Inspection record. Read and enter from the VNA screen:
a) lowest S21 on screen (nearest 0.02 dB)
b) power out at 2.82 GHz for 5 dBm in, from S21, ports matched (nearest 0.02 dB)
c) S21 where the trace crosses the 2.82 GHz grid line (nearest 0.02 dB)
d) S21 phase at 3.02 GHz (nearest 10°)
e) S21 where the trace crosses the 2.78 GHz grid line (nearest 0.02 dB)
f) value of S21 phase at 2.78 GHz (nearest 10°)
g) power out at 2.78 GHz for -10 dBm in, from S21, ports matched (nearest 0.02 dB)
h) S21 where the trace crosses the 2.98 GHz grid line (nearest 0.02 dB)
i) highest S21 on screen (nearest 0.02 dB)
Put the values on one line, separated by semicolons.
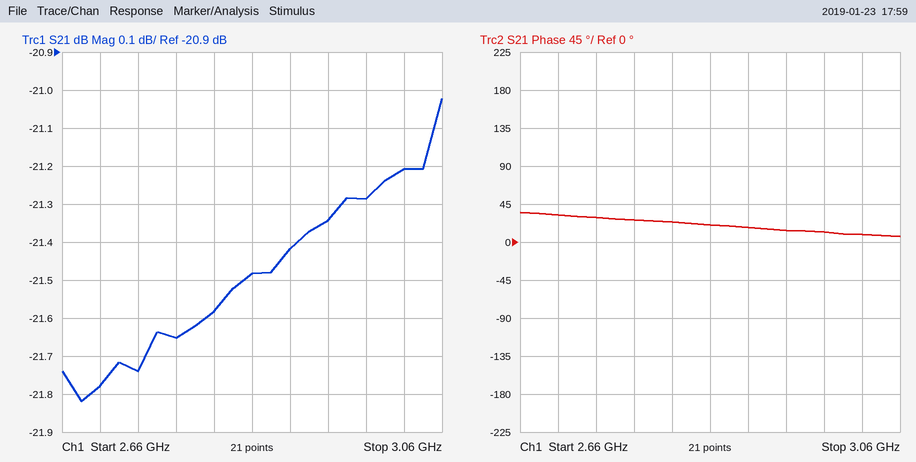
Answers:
-21.82 dB; -16.58 dBm; -21.58 dB; 10°; -21.66 dB; 30°; -31.66 dBm; -21.28 dB; -21.02 dB
